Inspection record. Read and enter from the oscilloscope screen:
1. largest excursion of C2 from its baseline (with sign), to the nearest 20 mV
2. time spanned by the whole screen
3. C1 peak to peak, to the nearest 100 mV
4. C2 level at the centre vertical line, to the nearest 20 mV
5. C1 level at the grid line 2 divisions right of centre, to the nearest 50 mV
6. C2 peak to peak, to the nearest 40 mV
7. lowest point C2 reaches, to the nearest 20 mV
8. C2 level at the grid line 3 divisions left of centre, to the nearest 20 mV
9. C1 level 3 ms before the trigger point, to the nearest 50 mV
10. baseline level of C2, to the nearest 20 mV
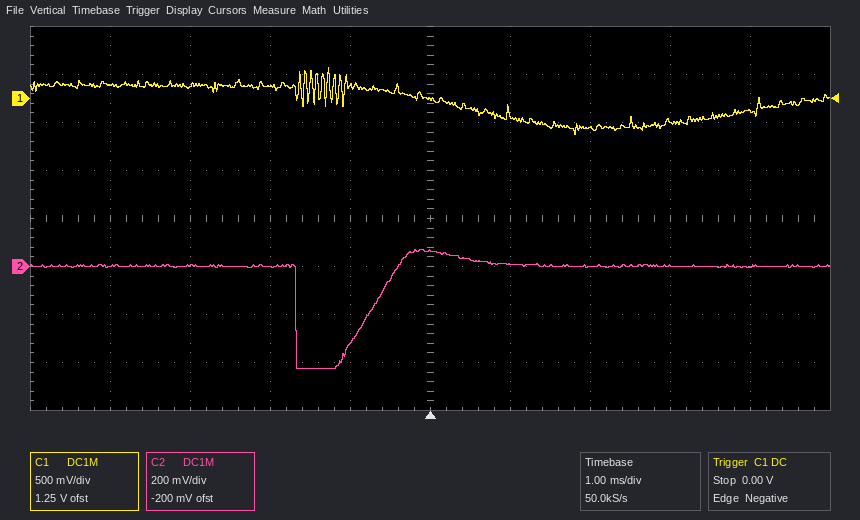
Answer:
-420 mV
10 ms
700 mV
60 mV
-300 mV
480 mV
-420 mV
0 mV
150 mV
0 mV
